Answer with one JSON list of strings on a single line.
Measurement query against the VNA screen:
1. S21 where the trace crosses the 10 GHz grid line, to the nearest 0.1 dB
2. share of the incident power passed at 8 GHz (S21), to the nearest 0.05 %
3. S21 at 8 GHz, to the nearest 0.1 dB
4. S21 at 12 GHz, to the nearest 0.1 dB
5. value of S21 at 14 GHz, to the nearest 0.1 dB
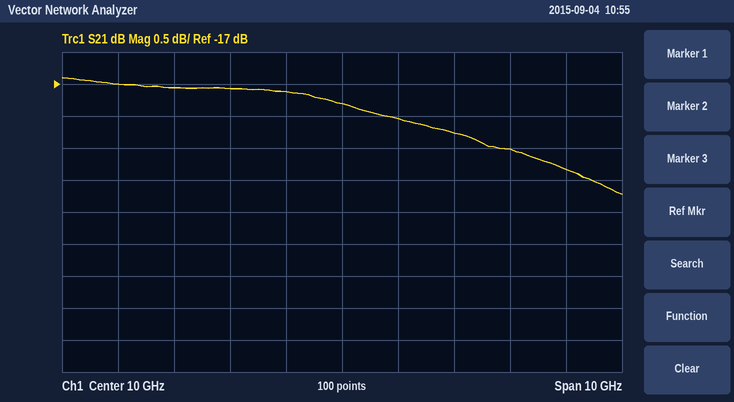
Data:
["-17.3 dB", "1.95 %", "-17.1 dB", "-17.8 dB", "-18.3 dB"]
